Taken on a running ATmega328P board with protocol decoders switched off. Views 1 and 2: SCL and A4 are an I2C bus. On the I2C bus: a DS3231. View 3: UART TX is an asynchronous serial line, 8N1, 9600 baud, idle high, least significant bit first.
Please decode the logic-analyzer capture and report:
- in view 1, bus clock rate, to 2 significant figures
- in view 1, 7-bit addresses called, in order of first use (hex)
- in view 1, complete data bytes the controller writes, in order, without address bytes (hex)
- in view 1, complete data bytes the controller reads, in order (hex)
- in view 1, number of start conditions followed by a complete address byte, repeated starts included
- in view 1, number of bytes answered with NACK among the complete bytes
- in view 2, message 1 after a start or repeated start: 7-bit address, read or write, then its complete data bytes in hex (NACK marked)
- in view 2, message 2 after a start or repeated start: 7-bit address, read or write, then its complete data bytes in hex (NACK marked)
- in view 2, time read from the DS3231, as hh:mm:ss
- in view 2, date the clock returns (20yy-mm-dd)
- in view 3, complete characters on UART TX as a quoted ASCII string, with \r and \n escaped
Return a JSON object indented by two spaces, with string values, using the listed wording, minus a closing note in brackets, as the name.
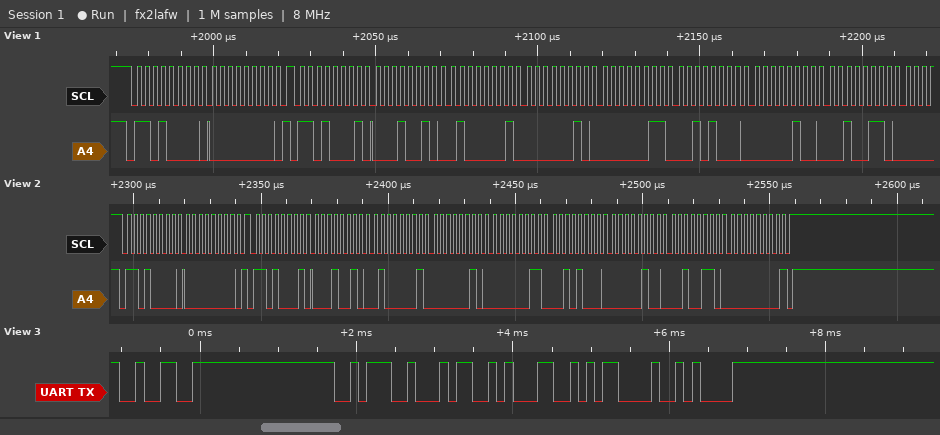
{
  "in view 1, bus clock rate, to 2 significant figures": "400 kHz",
  "in view 1, 7-bit addresses called, in order of first use": "0x68",
  "in view 1, complete data bytes the controller writes, in order, without address bytes": "00",
  "in view 1, complete data bytes the controller reads, in order": "12 41 02 03 28 04 26",
  "in view 1, number of start conditions followed by a complete address byte, repeated starts included": "2",
  "in view 1, number of bytes answered with NACK among the complete bytes": "0",
  "in view 2, message 1 after a start or repeated start: 7-bit address, read or write, then its complete data bytes in hex": "0x68 write: 00",
  "in view 2, message 2 after a start or repeated start: 7-bit address, read or write, then its complete data bytes in hex": "0x68 read: 12 41 02 03 28 04 26 00 NACK",
  "in view 2, time read from the DS3231, as hh:mm:ss": "02:41:12",
  "in view 2, date the clock returns": "2026-04-28",
  "in view 3, complete characters on UART TX as a quoted ASCII string, with \\r and \\n escaped": "\"2:41\\r\\n\""
}
